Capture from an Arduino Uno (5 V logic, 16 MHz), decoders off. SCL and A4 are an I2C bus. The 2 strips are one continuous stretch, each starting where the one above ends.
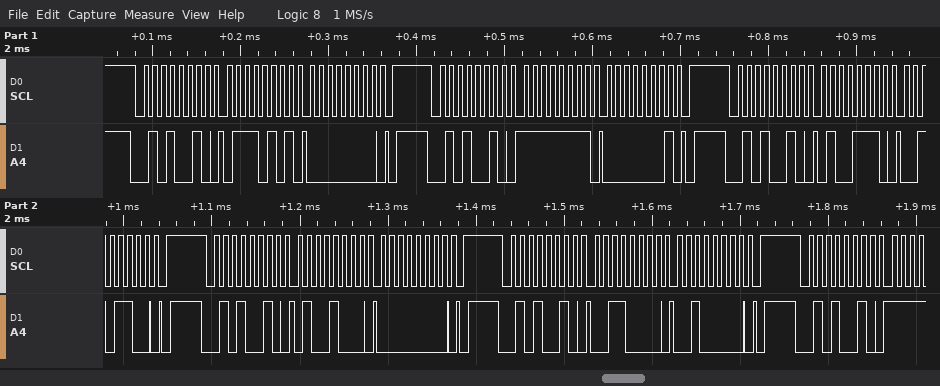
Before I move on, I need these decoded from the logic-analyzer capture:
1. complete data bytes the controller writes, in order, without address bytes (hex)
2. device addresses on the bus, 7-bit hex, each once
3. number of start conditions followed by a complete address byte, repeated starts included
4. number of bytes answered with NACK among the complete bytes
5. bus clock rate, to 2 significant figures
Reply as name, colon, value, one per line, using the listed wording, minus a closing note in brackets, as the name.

complete data bytes the controller writes, in order, without address bytes: 75 00 FF 01 4E 2C 48 00 30 20
device addresses on the bus, 7-bit hex, each once: 0x29
number of start conditions followed by a complete address byte, repeated starts included: 6
number of bytes answered with NACK among the complete bytes: 0
bus clock rate, to 2 significant figures: 100 kHz
